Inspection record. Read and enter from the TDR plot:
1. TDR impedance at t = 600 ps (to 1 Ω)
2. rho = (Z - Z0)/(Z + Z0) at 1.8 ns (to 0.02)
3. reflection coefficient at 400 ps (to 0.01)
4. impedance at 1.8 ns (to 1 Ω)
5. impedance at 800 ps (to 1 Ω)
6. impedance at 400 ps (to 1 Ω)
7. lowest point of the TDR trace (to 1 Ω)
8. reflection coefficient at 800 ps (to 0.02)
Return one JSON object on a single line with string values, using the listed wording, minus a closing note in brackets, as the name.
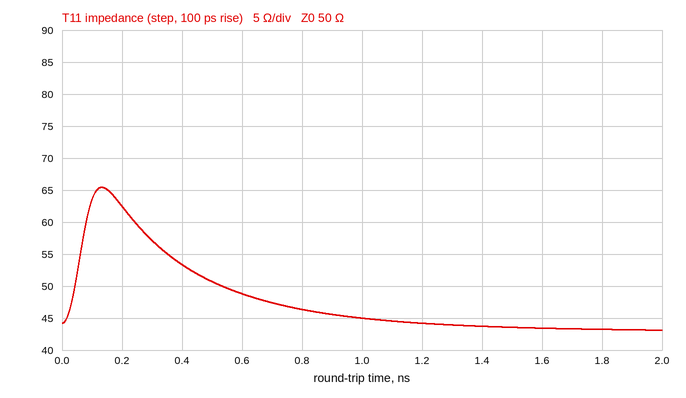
{"TDR impedance at t = 600 ps": "49 Ω", "rho = (Z - Z0)/(Z + Z0) at 1.8 ns": "-0.08", "reflection coefficient at 400 ps": "+0.03", "impedance at 1.8 ns": "43 Ω", "impedance at 800 ps": "46 Ω", "impedance at 400 ps": "53 Ω", "lowest point of the TDR trace": "43 Ω", "reflection coefficient at 800 ps": "-0.04"}
